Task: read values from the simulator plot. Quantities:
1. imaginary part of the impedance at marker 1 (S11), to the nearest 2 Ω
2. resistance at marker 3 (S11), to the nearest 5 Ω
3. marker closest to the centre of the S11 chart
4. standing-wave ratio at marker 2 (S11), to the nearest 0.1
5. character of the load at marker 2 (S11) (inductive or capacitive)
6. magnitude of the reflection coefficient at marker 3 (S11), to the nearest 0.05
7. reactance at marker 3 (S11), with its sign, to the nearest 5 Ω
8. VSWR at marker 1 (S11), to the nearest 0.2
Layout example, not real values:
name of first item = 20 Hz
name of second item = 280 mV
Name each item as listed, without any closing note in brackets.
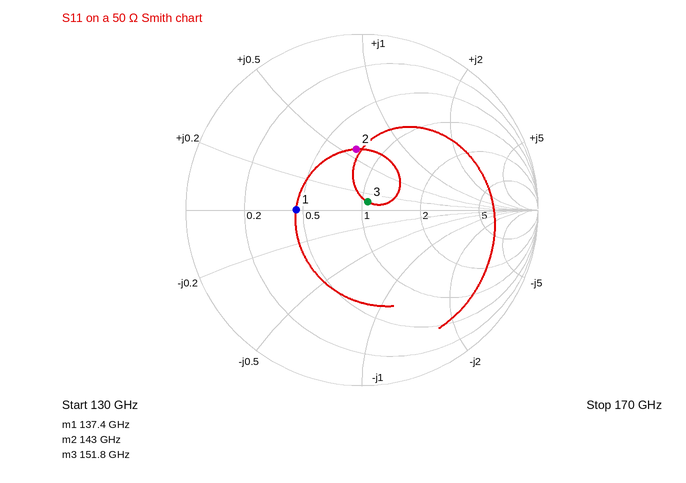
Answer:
imaginary part of the impedance at marker 1 (S11), to the nearest 2 Ω = 0 Ω
resistance at marker 3 (S11), to the nearest 5 Ω = 55 Ω
marker closest to the centre of the S11 chart = marker 3
standing-wave ratio at marker 2 (S11), to the nearest 0.1 = 2.1
character of the load at marker 2 (S11) = inductive
magnitude of the reflection coefficient at marker 3 (S11), to the nearest 0.05 = 0.05
reactance at marker 3 (S11), with its sign, to the nearest 5 Ω = +5 Ω
VSWR at marker 1 (S11), to the nearest 0.2 = 2.2
